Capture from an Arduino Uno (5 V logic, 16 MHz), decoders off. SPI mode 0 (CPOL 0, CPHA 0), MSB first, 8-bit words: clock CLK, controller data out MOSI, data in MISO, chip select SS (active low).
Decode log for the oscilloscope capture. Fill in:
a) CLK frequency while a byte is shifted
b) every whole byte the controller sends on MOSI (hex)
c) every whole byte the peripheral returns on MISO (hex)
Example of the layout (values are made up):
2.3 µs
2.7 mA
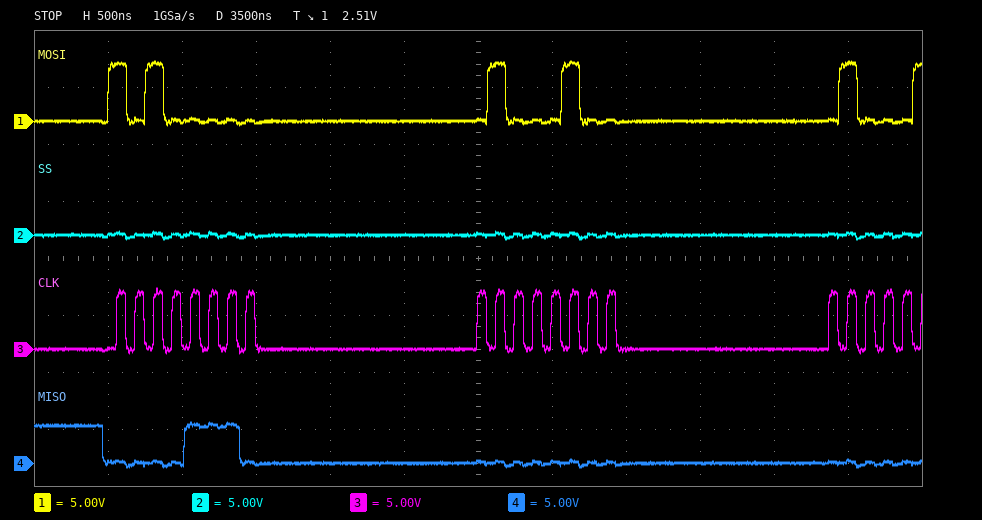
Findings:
8 MHz
A0 44
0E 00
